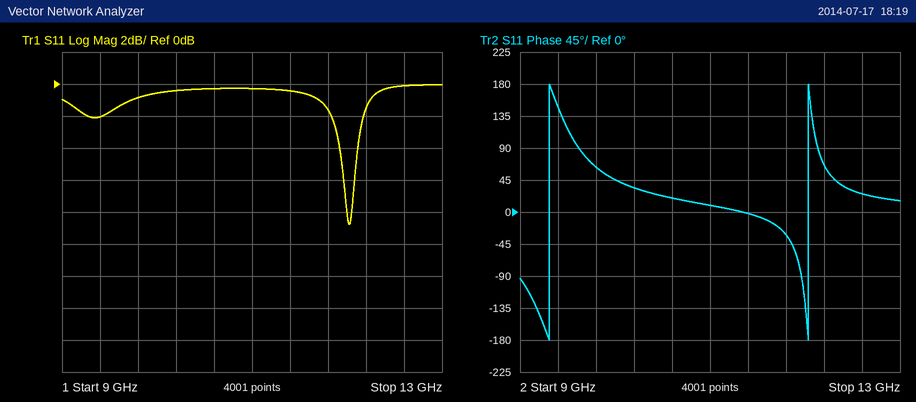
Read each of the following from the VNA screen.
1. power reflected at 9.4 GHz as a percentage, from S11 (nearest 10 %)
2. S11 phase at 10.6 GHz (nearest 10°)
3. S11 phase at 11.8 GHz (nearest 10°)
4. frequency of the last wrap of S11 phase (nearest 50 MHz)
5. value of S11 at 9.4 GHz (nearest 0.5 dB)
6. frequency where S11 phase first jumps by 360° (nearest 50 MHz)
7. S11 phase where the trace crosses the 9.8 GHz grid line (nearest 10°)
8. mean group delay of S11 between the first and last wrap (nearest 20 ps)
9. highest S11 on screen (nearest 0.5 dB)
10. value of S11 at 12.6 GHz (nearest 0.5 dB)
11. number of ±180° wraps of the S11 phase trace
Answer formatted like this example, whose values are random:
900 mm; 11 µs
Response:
60 %; 20°; -30°; 12.05 GHz; -2.0 dB; 9.30 GHz; 60°; 360 ps; 0.0 dB; 0.0 dB; 2
